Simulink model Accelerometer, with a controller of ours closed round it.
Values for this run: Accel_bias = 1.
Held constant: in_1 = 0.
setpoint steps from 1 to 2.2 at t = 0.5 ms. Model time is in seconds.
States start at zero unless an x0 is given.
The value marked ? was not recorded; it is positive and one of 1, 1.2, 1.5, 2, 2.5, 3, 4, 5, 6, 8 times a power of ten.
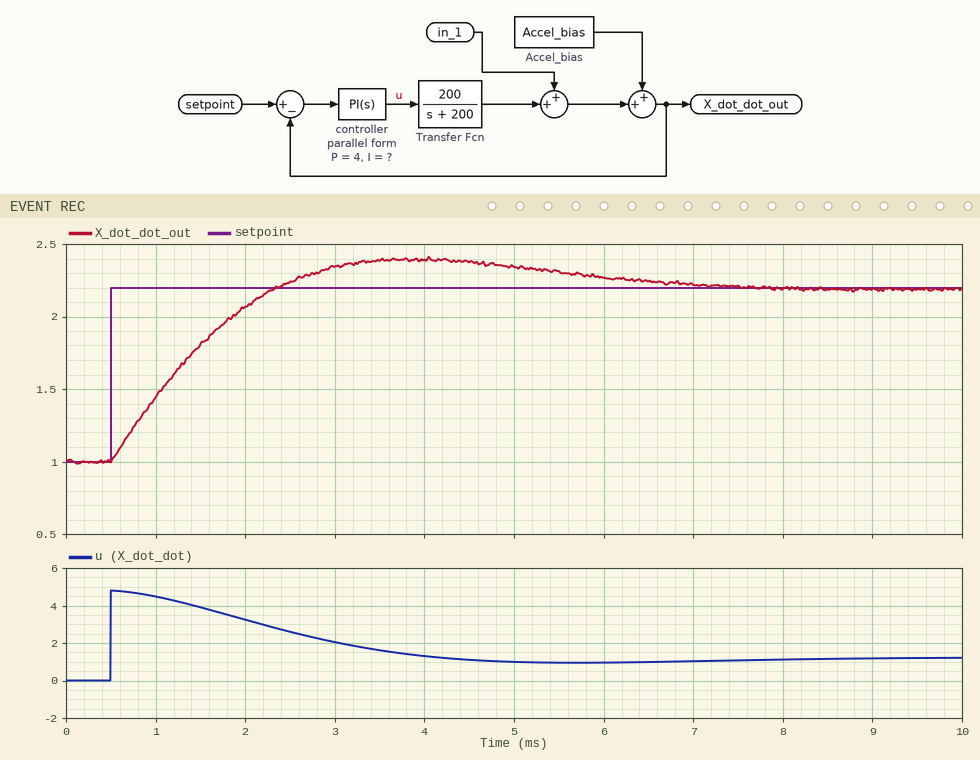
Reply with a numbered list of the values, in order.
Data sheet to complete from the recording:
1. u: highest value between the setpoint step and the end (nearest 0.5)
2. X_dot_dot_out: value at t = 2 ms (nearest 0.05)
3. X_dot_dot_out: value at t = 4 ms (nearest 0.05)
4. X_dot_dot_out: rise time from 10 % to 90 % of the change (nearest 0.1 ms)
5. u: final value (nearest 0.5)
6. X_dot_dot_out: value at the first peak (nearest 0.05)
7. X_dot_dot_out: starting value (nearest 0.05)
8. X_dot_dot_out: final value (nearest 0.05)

1. 5.0
2. 2.05
3. 2.40
4. 1.4 ms
5. 1.0
6. 2.40
7. 1.00
8. 2.20
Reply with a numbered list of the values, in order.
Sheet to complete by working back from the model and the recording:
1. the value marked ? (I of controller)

1. 3000
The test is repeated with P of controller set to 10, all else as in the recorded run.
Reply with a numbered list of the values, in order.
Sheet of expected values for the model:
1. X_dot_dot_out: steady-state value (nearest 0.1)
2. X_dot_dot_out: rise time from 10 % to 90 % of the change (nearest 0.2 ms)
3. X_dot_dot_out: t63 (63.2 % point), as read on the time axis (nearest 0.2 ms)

1. 2.2
2. 1.0 ms
3. 1.0 ms
